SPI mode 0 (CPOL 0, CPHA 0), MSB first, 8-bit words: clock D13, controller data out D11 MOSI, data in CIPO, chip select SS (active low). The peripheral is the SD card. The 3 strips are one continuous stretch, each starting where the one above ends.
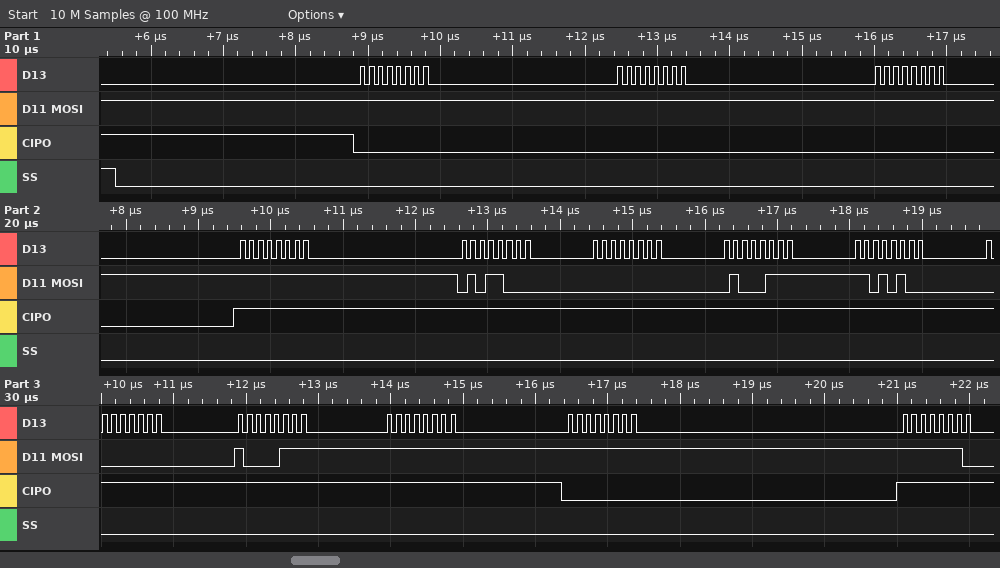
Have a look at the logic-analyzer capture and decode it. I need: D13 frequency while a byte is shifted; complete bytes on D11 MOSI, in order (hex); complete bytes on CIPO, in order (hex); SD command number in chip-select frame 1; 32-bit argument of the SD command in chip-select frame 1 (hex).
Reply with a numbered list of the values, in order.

1. 8 MHz
2. FF FF FF FF 58 00 47 D4 00 87 FF FF FE
3. 00 00 00 FF FF FF FF FF FF FF FF 00 FF
4. CMD24
5. 0x0047D400
